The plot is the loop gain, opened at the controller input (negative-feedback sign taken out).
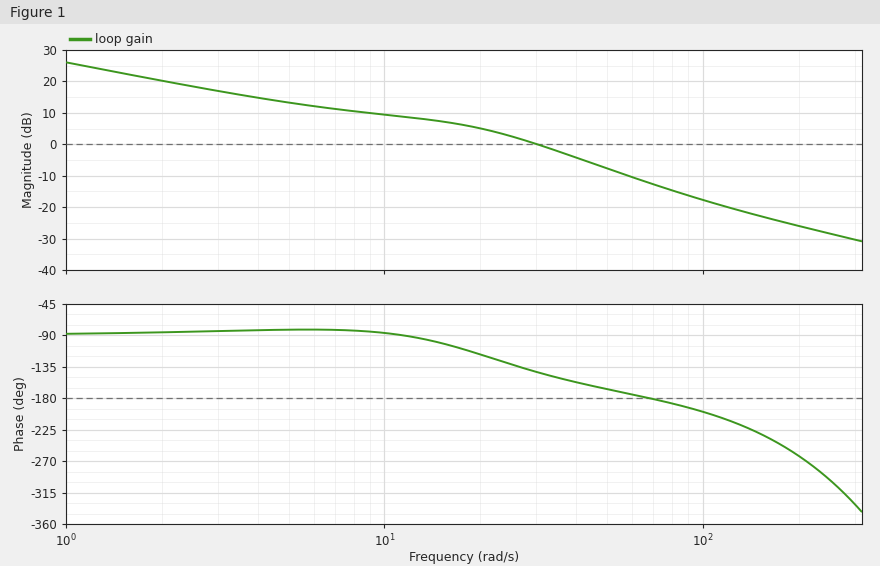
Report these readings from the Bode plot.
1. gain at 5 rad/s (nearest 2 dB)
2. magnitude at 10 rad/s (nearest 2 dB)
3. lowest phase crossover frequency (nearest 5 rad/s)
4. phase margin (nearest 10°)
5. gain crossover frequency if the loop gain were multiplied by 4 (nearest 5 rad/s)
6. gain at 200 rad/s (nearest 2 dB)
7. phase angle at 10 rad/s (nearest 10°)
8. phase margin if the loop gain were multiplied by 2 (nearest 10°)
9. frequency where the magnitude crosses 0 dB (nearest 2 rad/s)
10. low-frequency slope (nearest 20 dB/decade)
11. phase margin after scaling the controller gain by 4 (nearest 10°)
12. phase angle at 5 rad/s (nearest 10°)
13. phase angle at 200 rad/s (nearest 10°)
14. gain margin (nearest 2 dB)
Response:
14 dB
10 dB
70 rad/s
40°
65 rad/s
-26 dB
-90°
20°
30 rad/s
-20 dB/decade
0°
-80°
-260°
12 dB
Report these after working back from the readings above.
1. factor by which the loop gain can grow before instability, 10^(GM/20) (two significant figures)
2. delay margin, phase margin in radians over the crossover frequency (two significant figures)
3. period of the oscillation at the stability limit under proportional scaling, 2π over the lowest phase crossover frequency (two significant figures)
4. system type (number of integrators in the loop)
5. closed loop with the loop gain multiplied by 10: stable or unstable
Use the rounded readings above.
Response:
4.0
0.023 s
0.090 s
1
unstable
